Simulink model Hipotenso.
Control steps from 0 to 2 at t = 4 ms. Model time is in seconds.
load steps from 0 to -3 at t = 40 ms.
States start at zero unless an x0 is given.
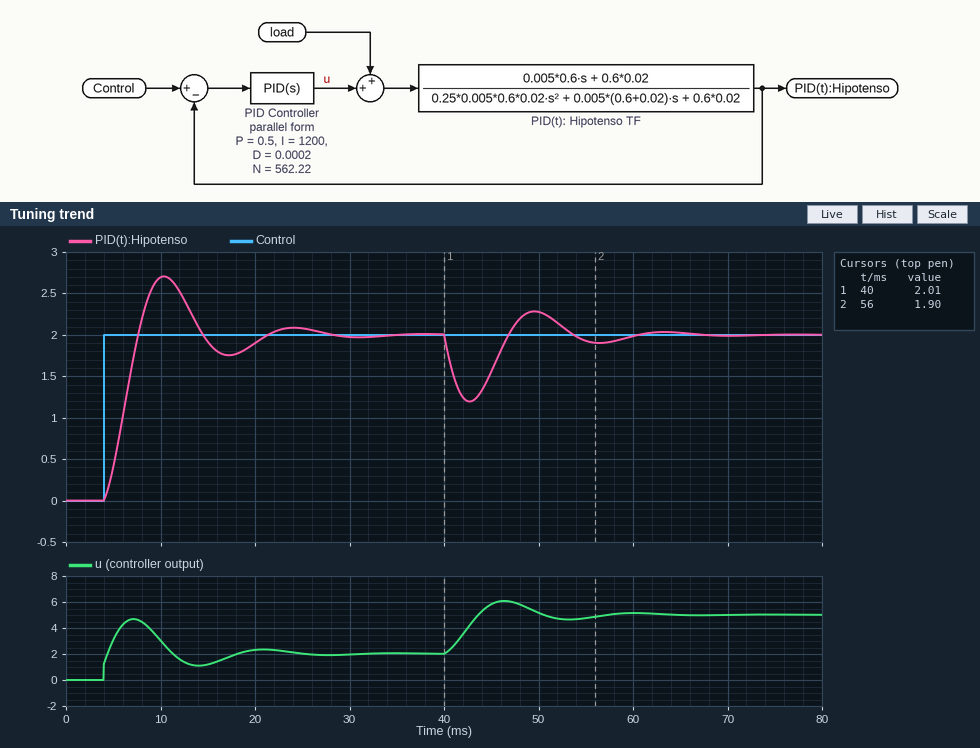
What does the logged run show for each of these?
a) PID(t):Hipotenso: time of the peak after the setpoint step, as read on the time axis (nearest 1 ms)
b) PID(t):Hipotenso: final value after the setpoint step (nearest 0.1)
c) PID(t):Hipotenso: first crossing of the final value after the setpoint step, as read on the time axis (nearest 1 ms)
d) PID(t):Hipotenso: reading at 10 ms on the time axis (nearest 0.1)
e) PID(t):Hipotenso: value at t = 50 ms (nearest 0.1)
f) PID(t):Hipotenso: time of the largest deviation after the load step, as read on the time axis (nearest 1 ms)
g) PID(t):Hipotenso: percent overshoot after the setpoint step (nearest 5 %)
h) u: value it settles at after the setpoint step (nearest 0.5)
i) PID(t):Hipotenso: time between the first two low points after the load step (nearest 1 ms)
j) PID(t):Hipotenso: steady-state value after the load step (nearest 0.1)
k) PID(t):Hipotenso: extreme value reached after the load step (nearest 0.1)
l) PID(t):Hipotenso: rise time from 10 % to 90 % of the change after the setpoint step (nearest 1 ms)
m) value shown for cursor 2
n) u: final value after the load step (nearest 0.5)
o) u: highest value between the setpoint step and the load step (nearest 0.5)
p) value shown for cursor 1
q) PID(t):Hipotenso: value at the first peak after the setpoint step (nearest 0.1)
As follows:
10 ms
2.0
8 ms
2.7
2.3
43 ms
35 %
2.0
14 ms
2.0
1.2
3 ms
1.90
5.0
4.5
2.01
2.7
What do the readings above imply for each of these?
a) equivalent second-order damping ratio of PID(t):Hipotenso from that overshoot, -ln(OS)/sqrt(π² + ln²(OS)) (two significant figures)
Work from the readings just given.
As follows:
0.32
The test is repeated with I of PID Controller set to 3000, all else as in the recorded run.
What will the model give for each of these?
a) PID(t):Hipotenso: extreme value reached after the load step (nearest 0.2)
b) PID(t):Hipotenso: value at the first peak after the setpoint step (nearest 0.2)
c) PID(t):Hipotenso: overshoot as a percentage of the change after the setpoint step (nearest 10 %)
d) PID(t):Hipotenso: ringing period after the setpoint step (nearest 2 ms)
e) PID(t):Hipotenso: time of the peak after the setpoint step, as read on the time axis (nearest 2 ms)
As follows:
1.4
3.0
50 %
8 ms
8 ms
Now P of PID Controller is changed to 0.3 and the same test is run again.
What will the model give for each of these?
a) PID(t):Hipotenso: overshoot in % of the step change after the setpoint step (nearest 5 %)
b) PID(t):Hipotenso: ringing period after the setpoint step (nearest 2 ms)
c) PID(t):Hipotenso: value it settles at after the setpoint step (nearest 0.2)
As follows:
40 %
14 ms
2.0
